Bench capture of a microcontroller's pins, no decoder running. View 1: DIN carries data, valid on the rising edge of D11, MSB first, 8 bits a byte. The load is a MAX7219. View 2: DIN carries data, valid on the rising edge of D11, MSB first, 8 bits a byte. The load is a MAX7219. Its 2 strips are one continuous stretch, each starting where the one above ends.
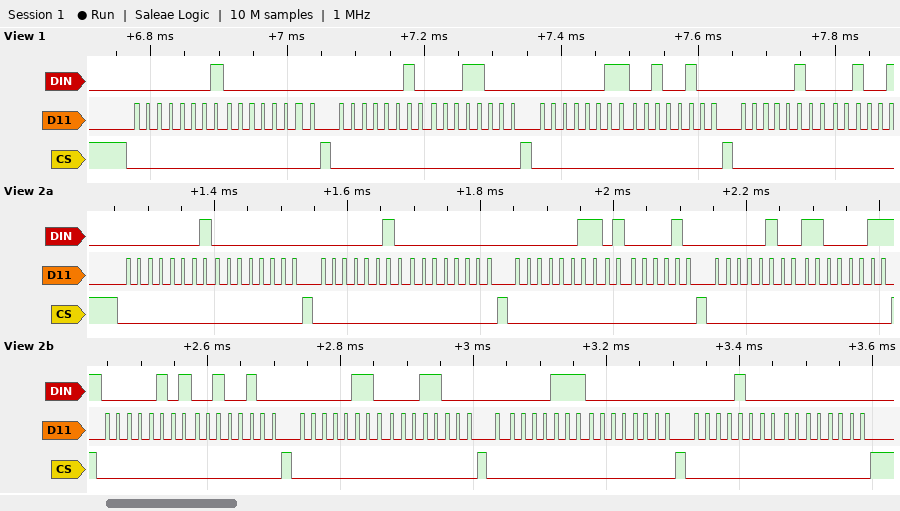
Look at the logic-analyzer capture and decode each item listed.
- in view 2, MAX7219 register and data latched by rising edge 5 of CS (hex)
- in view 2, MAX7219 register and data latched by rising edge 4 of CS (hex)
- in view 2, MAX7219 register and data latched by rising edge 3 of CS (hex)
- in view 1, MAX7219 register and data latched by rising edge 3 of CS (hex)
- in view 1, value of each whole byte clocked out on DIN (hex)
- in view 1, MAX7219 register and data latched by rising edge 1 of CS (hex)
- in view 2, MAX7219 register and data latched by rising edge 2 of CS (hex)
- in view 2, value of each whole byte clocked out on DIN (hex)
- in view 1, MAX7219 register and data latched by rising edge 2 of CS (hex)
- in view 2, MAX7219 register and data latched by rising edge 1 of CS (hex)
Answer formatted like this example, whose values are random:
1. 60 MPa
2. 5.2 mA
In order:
1. register 0x5, data 0x24
2. register 0x4, data 0xC3
3. register 0x3, data 0x42
4. register 0x3, data 0x24
5. 0x01 0x00 0x02 0x18 0x03 0x24 0x04
6. register 0x1, data 0x00
7. register 0x2, data 0x00
8. 01 00 02 00 03 42 04 C3 05 24 06 18 07 00 08 00
9. register 0x2, data 0x18
10. register 0x1, data 0x00
